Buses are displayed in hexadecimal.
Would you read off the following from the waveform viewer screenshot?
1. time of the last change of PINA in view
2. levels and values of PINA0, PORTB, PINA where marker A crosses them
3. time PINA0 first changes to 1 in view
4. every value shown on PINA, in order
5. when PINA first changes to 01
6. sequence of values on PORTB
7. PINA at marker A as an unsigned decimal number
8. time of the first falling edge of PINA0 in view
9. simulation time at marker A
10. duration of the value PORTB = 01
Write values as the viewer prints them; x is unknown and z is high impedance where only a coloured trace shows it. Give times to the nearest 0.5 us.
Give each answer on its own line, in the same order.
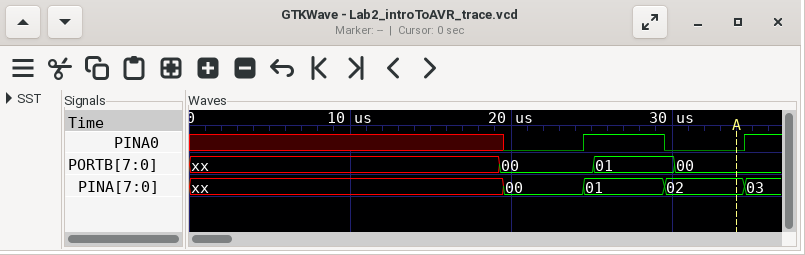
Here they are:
34.5 us
PINA0=0, PORTB=00, PINA=02
24.5 us
xx, 00, 01, 02, 03
24.5 us
xx, 00, 01, 00
2
29.5 us
34 us
5 us
